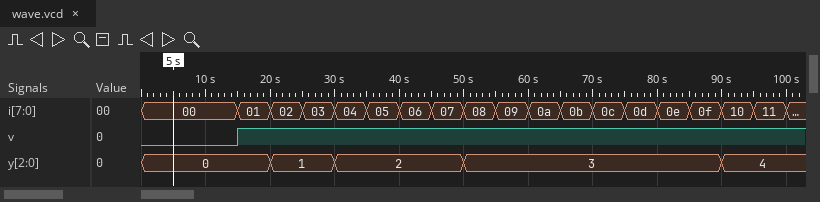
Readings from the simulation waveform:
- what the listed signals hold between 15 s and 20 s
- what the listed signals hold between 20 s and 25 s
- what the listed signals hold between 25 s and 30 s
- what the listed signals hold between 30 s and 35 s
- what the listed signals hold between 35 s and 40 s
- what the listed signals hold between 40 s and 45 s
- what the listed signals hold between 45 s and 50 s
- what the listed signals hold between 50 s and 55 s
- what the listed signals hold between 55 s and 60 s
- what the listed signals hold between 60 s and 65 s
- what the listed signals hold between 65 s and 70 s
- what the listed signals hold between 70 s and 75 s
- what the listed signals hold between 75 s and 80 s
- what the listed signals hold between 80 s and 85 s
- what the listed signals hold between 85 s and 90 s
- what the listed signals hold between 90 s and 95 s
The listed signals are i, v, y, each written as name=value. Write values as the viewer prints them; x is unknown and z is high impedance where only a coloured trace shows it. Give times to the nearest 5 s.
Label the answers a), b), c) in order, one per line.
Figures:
a) i=01, v=1, y=0
b) i=02, v=1, y=1
c) i=03, v=1, y=1
d) i=04, v=1, y=2
e) i=05, v=1, y=2
f) i=06, v=1, y=2
g) i=07, v=1, y=2
h) i=08, v=1, y=3
i) i=09, v=1, y=3
j) i=0a, v=1, y=3
k) i=0b, v=1, y=3
l) i=0c, v=1, y=3
m) i=0d, v=1, y=3
n) i=0e, v=1, y=3
o) i=0f, v=1, y=3
p) i=10, v=1, y=4
